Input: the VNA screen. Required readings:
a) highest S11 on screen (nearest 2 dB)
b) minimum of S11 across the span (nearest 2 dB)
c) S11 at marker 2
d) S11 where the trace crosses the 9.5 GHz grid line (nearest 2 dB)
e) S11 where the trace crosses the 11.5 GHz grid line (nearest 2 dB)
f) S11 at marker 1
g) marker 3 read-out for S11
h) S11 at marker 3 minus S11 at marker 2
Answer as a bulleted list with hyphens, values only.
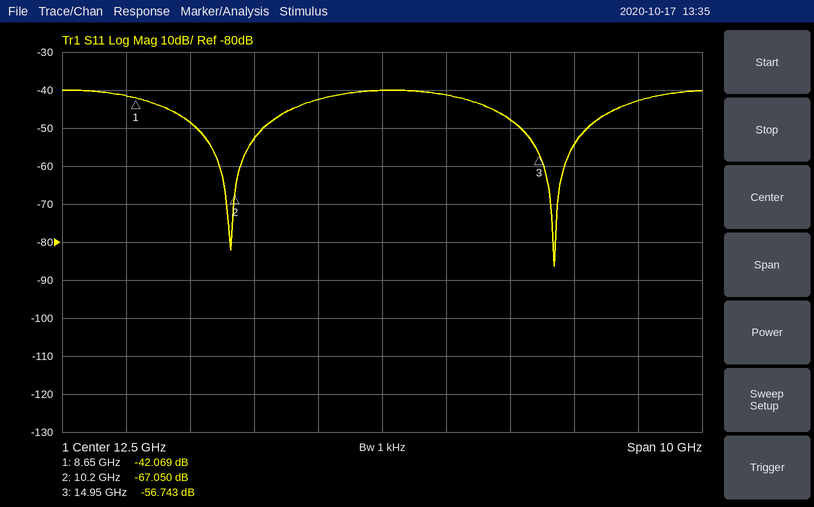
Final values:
- -40 dB
- -86 dB
- -67.050 dB
- -48 dB
- -42 dB
- -42.069 dB
- -56.743 dB
- 10.307 dB
